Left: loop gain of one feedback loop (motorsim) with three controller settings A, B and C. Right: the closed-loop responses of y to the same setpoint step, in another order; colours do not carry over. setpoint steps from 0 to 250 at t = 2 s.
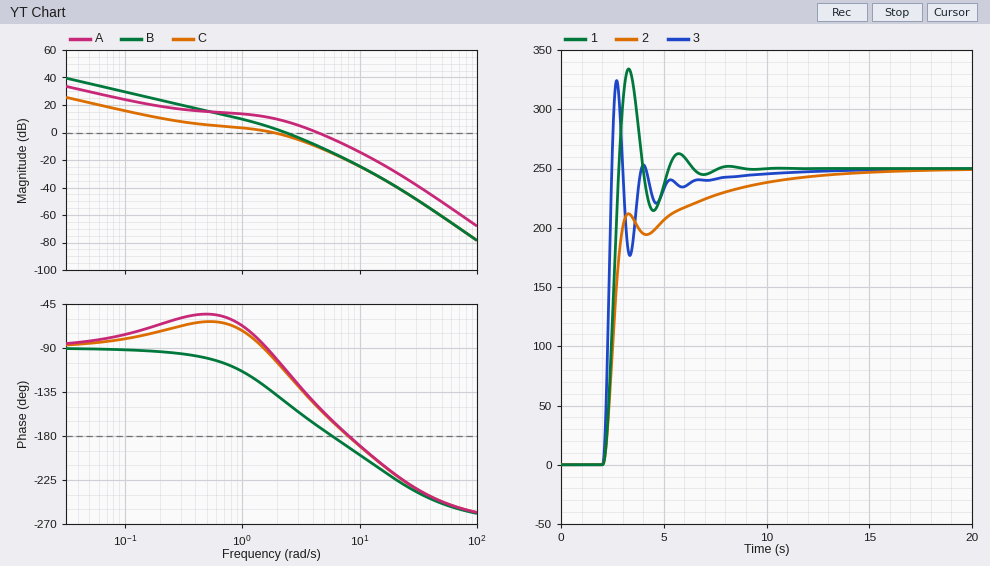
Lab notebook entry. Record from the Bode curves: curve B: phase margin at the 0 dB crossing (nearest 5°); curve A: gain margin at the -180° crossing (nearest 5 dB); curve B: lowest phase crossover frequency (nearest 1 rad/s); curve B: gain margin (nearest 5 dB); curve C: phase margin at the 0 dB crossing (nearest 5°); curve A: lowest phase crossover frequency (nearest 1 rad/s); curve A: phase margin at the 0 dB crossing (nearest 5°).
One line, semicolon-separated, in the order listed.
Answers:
35°; 10 dB; 6 rad/s; 15 dB; 80°; 8 rad/s; 30°
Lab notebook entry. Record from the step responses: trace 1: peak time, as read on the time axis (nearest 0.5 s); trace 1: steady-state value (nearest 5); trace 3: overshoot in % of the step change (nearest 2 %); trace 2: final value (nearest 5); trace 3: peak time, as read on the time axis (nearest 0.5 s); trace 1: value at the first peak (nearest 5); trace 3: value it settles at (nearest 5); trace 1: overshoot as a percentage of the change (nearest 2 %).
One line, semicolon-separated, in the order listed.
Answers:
3.5 s; 250; 30 %; 250; 2.5 s; 335; 250; 34 %
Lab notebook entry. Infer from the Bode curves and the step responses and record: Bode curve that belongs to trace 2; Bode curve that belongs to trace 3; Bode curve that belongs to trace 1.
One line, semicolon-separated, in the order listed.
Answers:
C; A; B
